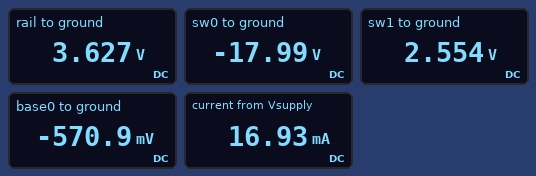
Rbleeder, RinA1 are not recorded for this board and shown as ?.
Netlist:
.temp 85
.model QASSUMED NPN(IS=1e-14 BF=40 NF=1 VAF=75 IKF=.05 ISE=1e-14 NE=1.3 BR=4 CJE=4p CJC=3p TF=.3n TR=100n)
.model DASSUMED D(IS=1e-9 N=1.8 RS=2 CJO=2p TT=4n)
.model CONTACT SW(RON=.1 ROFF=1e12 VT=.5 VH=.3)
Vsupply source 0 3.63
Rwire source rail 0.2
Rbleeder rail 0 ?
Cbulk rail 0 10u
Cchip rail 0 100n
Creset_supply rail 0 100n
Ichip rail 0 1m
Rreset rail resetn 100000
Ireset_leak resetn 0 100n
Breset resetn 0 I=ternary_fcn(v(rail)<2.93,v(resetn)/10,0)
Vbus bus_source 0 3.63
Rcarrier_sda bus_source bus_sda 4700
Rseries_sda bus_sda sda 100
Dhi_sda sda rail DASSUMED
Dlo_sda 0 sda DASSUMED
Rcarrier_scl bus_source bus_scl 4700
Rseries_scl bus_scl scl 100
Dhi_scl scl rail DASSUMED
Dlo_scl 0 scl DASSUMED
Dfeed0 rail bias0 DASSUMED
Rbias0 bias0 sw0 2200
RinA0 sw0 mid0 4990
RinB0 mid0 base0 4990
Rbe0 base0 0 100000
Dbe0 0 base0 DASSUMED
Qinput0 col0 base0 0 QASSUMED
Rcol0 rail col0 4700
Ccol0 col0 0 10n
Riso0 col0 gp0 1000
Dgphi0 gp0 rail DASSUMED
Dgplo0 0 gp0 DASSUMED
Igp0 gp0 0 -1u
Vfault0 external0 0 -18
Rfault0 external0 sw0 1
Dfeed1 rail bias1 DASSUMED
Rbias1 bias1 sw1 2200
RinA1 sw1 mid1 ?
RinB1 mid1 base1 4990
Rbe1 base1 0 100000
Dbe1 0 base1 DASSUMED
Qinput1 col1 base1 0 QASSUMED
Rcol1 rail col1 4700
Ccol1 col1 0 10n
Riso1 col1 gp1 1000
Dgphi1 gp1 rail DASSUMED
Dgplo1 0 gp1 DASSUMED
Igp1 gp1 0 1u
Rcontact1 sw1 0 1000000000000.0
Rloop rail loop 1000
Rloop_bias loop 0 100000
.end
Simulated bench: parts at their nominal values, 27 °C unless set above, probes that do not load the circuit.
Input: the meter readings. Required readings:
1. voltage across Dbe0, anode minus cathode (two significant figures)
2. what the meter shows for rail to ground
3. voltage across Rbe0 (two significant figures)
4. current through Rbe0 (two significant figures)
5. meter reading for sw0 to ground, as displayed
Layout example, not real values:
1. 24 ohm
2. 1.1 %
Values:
1. 570 mV
2. 3.627 V
3. 570 mV
4. 5.7 µA
5. -17.99 V
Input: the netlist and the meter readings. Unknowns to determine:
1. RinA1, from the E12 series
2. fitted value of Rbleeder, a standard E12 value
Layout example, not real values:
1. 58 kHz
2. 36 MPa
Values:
1. 2.2 kΩ
2. 680 Ω
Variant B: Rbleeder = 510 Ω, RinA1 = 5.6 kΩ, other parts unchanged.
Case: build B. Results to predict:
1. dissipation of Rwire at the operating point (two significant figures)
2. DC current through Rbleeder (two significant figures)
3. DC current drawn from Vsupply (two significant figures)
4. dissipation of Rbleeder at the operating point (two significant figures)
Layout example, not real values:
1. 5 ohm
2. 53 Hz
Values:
1. 69 µW
2. 7.1 mA
3. 19 mA
4. 26 mW
